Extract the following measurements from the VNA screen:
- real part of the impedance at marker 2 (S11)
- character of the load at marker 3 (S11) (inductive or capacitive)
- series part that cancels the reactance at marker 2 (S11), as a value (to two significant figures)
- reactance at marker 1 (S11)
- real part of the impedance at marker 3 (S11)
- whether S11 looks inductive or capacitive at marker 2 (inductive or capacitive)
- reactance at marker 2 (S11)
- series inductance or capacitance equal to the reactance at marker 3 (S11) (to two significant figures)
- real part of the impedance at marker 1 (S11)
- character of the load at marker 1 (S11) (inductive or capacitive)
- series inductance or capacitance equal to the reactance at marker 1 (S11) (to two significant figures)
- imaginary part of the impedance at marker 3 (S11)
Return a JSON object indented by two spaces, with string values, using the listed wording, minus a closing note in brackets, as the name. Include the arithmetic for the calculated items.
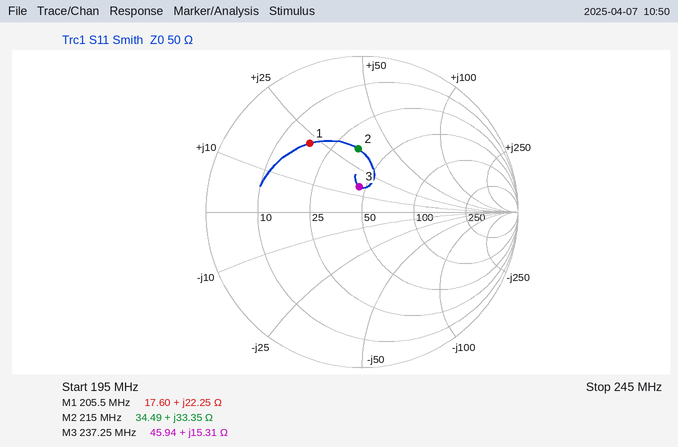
{
  "real part of the impedance at marker 2": "34.49 Ω",
  "character of the load at marker 3 (S11)": "inductive",
  "series part that cancels the reactance at marker 2 (S11), as a value": "C = 1/(2π × 215 MHz × 33.35 Ω) ≈ 22 pF",
  "reactance at marker 1": "+22.25 Ω",
  "real part of the impedance at marker 3": "45.94 Ω",
  "whether S11 looks inductive or capacitive at marker 2": "inductive",
  "reactance at marker 2": "+33.35 Ω",
  "series inductance or capacitance equal to the reactance at marker 3 (S11)": "L = 15.31 Ω/(2π × 237.25 MHz) ≈ 10 nH",
  "real part of the impedance at marker 1": "17.60 Ω",
  "character of the load at marker 1 (S11)": "inductive",
  "series inductance or capacitance equal to the reactance at marker 1 (S11)": "L = 22.25 Ω/(2π × 205.5 MHz) ≈ 17 nH",
  "imaginary part of the impedance at marker 3": "+15.31 Ω"
}
